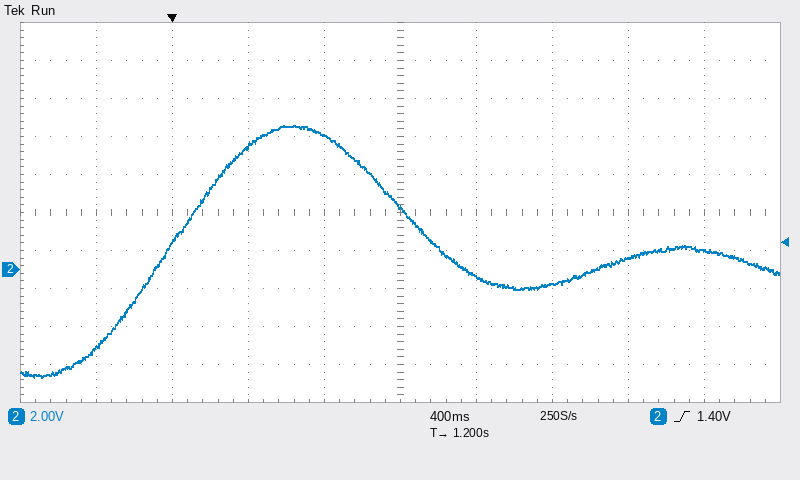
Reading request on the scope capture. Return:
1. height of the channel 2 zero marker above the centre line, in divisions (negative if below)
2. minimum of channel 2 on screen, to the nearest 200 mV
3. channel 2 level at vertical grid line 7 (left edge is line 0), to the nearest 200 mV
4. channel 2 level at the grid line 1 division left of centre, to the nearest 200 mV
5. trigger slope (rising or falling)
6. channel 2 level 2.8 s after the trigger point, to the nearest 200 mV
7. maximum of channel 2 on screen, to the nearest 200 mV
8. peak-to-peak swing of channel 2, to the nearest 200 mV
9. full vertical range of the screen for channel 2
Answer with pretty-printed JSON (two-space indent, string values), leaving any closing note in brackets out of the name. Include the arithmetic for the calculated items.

{
  "height of the channel 2 zero marker above the centre line, in divisions": "-1.5 div",
  "minimum of channel 2 on screen, to the nearest 200 mV": "-5.6 V",
  "channel 2 level at vertical grid line 7 (left edge is line 0), to the nearest 200 mV": "-800 mV",
  "channel 2 level at the grid line 1 division left of centre, to the nearest 200 mV": "7.0 V",
  "trigger slope": "rising",
  "channel 2 level 2.8 s after the trigger point, to the nearest 200 mV": "1.0 V",
  "maximum of channel 2 on screen, to the nearest 200 mV": "7.6 V",
  "peak-to-peak swing of channel 2, to the nearest 200 mV": "7.6 V − (-5.6 V) = 13.2 V",
  "full vertical range of the screen for channel 2": "20 V"
}
